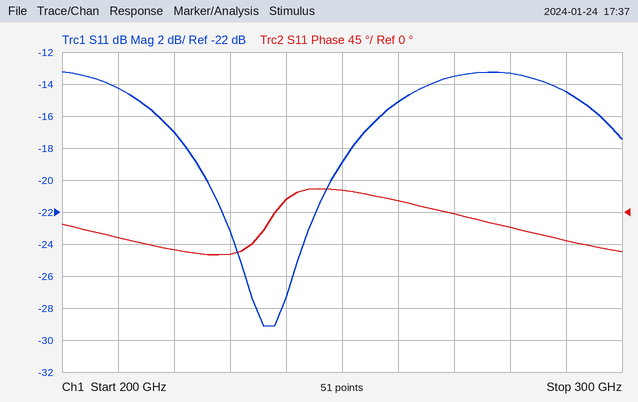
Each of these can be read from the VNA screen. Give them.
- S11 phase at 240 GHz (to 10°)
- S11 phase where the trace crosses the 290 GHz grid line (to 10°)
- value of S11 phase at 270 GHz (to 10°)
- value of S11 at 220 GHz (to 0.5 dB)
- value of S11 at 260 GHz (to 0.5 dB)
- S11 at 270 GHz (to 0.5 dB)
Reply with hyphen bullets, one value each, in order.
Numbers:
- 20°
- -40°
- 0°
- -17.0 dB
- -15.0 dB
- -13.5 dB
